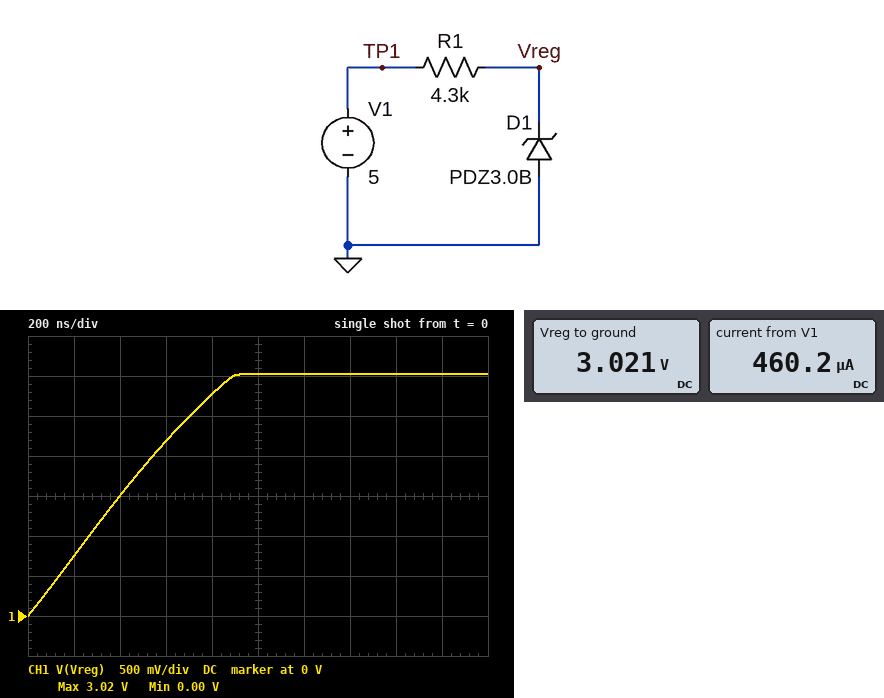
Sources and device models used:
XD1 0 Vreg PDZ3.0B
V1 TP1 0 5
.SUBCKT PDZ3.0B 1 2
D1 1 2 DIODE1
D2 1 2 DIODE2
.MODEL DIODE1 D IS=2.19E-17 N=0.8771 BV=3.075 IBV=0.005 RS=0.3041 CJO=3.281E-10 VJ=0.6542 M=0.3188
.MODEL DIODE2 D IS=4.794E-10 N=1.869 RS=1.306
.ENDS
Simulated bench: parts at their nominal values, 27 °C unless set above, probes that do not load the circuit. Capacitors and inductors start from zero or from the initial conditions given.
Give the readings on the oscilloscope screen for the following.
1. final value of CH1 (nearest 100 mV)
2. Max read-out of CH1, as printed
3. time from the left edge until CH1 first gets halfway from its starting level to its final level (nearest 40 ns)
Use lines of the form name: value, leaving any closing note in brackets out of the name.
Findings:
final value of CH1: 3.0 V
Max read-out of CH1, as printed: 3.02 V
time from the left edge until CH1 first gets halfway from its starting level to its final level: 400 ns
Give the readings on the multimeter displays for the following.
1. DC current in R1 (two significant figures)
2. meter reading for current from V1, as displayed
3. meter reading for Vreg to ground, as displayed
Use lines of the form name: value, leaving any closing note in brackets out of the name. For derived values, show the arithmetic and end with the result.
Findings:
DC current in R1: (5 V - 3.021 V) / 4.3 kΩ = 460 µA
meter reading for current from V1, as displayed: 460.2 µA
meter reading for Vreg to ground, as displayed: 3.021 V
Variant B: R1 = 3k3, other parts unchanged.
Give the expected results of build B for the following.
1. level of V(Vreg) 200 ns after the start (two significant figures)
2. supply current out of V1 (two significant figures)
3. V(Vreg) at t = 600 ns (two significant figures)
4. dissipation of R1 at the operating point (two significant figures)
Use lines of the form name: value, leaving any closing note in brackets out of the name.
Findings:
level of V(Vreg) 200 ns after the start: 980 mV
supply current out of V1: 600 µA
V(Vreg) at t = 600 ns: 2.7 V
dissipation of R1 at the operating point: 1.2 mW
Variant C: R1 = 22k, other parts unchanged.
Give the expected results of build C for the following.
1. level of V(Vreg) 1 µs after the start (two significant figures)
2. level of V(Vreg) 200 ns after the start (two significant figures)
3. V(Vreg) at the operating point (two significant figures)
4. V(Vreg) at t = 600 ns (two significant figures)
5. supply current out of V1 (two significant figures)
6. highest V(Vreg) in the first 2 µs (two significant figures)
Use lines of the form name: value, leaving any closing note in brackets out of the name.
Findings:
level of V(Vreg) 1 µs after the start: 730 mV
level of V(Vreg) 200 ns after the start: 140 mV
V(Vreg) at the operating point: 3.0 V
V(Vreg) at t = 600 ns: 430 mV
supply current out of V1: 92 µA
highest V(Vreg) in the first 2 µs: 1.5 V
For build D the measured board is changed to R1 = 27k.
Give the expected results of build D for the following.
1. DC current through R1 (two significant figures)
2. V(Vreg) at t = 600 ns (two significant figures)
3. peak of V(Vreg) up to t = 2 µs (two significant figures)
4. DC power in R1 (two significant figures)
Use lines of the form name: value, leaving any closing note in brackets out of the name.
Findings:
DC current through R1: 75 µA
V(Vreg) at t = 600 ns: 350 mV
peak of V(Vreg) up to t = 2 µs: 1.2 V
DC power in R1: 150 µW
